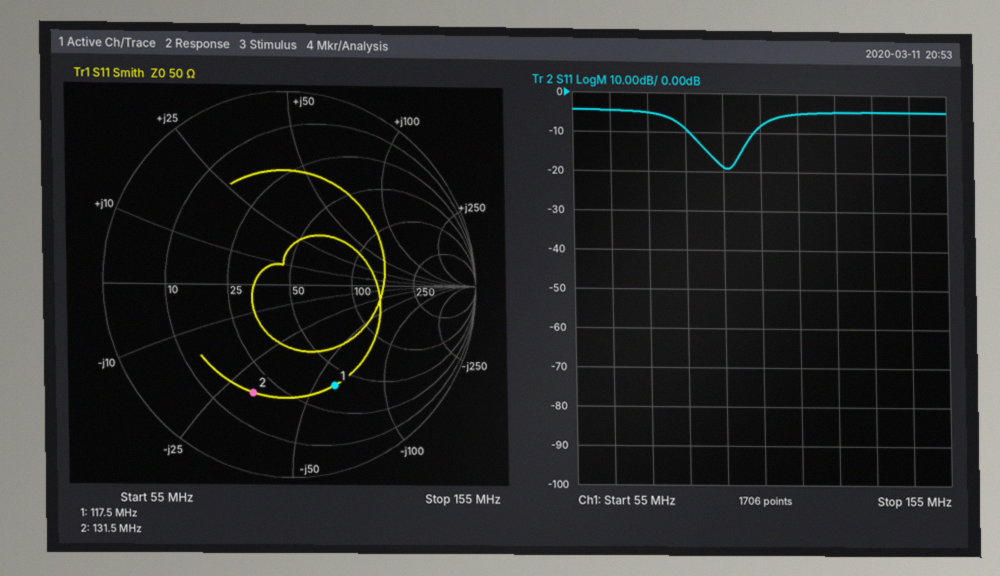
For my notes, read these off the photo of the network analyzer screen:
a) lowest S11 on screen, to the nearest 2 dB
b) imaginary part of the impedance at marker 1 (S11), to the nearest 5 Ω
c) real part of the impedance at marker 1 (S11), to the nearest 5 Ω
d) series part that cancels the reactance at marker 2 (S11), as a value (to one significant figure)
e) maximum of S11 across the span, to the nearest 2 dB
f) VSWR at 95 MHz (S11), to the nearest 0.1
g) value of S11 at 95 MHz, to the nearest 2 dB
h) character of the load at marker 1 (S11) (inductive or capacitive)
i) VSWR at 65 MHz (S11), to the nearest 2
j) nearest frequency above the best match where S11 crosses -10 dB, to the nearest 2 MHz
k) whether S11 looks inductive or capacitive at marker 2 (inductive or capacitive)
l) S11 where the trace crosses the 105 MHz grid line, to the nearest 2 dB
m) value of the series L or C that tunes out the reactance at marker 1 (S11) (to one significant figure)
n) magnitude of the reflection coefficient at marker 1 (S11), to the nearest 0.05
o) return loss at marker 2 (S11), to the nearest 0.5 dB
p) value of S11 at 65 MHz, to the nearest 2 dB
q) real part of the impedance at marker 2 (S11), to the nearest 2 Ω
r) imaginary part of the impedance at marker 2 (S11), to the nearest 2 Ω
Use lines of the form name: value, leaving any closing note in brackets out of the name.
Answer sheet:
lowest S11 on screen, to the nearest 2 dB: -20 dB
imaginary part of the impedance at marker 1 (S11), to the nearest 5 Ω: -60 Ω
real part of the impedance at marker 1 (S11), to the nearest 5 Ω: 40 Ω
series part that cancels the reactance at marker 2 (S11), as a value: 40 nH
maximum of S11 across the span, to the nearest 2 dB: -4 dB
VSWR at 95 MHz (S11), to the nearest 0.1: 1.3
value of S11 at 95 MHz, to the nearest 2 dB: -18 dB
character of the load at marker 1 (S11): capacitive
VSWR at 65 MHz (S11), to the nearest 2: 4
nearest frequency above the best match where S11 crosses -10 dB, to the nearest 2 MHz: 104 MHz
whether S11 looks inductive or capacitive at marker 2: capacitive
S11 where the trace crosses the 105 MHz grid line, to the nearest 2 dB: -8 dB
value of the series L or C that tunes out the reactance at marker 1 (S11): 80 nH
magnitude of the reflection coefficient at marker 1 (S11), to the nearest 0.05: 0.55
return loss at marker 2 (S11), to the nearest 0.5 dB: 4.5 dB
value of S11 at 65 MHz, to the nearest 2 dB: -4 dB
real part of the impedance at marker 2 (S11), to the nearest 2 Ω: 18 Ω
imaginary part of the impedance at marker 2 (S11), to the nearest 2 Ω: -32 Ω
